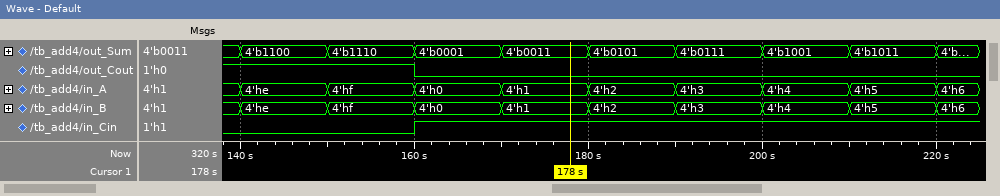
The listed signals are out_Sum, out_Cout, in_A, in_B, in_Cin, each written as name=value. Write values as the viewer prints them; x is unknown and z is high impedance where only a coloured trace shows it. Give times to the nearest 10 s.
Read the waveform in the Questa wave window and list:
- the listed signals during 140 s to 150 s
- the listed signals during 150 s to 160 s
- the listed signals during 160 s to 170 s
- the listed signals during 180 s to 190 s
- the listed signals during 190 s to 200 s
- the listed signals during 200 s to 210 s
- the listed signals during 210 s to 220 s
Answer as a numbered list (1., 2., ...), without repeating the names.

1. out_Sum=4'b1100, out_Cout=1, in_A=4'he, in_B=4'he, in_Cin=0
2. out_Sum=4'b1110, out_Cout=1, in_A=4'hf, in_B=4'hf, in_Cin=0
3. out_Sum=4'b0001, out_Cout=0, in_A=4'h0, in_B=4'h0, in_Cin=1
4. out_Sum=4'b0101, out_Cout=0, in_A=4'h2, in_B=4'h2, in_Cin=1
5. out_Sum=4'b0111, out_Cout=0, in_A=4'h3, in_B=4'h3, in_Cin=1
6. out_Sum=4'b1001, out_Cout=0, in_A=4'h4, in_B=4'h4, in_Cin=1
7. out_Sum=4'b1011, out_Cout=0, in_A=4'h5, in_B=4'h5, in_Cin=1
